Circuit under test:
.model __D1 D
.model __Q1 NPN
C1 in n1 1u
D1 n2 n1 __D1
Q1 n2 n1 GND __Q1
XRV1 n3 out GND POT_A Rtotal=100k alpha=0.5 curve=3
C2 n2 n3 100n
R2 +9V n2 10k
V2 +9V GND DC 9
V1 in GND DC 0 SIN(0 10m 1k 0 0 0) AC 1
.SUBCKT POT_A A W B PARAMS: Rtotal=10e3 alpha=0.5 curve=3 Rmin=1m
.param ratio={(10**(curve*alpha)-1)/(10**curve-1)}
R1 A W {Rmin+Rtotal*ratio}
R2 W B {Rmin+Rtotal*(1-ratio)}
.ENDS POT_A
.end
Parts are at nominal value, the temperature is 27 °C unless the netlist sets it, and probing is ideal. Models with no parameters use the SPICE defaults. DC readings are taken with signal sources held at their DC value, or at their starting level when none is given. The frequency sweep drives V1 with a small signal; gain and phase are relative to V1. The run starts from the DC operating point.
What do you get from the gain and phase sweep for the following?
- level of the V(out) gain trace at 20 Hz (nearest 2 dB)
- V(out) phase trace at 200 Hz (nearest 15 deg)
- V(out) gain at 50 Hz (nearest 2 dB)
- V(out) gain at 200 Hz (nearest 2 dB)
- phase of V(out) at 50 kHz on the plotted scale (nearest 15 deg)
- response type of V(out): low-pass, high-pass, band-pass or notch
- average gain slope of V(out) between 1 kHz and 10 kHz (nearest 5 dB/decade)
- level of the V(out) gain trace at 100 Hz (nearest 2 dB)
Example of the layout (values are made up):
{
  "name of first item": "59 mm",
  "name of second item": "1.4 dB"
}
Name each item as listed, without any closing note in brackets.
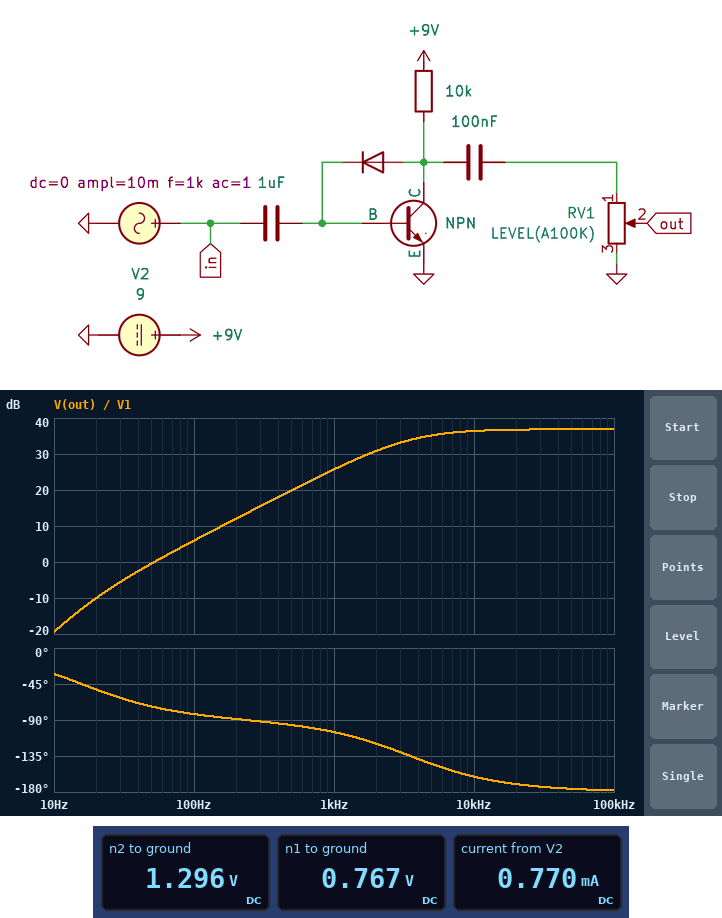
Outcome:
{
  "level of the V(out) gain trace at 20 Hz": "-10 dB",
  "V(out) phase trace at 200 Hz": "-90 deg",
  "V(out) gain at 50 Hz": "0 dB",
  "V(out) gain at 200 Hz": "12 dB",
  "phase of V(out) at 50 kHz on the plotted scale": "-180 deg",
  "response type of V(out): low-pass, high-pass, band-pass or notch": "high-pass",
  "average gain slope of V(out) between 1 kHz and 10 kHz": "10 dB/decade",
  "level of the V(out) gain trace at 100 Hz": "6 dB"
}
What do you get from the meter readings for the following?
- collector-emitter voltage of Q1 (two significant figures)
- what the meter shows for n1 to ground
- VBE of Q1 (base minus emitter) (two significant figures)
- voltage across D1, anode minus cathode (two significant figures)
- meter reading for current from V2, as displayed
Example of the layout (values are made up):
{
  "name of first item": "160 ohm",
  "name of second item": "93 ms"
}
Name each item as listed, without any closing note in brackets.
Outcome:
{
  "collector-emitter voltage of Q1": "1.3 V",
  "what the meter shows for n1 to ground": "0.767 V",
  "VBE of Q1 (base minus emitter)": "770 mV",
  "voltage across D1, anode minus cathode": "530 mV",
  "meter reading for current from V2, as displayed": "0.770 mA"
}
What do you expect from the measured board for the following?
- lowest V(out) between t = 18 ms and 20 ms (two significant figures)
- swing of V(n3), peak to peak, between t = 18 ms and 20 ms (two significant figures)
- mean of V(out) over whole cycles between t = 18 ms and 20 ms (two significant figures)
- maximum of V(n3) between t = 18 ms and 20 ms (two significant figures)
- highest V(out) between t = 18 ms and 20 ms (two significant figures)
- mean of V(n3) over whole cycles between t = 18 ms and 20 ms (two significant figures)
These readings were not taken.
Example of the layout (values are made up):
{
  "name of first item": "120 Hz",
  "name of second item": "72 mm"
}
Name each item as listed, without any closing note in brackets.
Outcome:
{
  "lowest V(out) between t = 18 ms and 20 ms": "-750 mV",
  "swing of V(n3), peak to peak, between t = 18 ms and 20 ms": "1.3 V",
  "mean of V(out) over whole cycles between t = 18 ms and 20 ms": "-77 mV",
  "maximum of V(n3) between t = 18 ms and 20 ms": "520 mV",
  "highest V(out) between t = 18 ms and 20 ms": "500 mV",
  "mean of V(n3) over whole cycles between t = 18 ms and 20 ms": "-79 mV"
}
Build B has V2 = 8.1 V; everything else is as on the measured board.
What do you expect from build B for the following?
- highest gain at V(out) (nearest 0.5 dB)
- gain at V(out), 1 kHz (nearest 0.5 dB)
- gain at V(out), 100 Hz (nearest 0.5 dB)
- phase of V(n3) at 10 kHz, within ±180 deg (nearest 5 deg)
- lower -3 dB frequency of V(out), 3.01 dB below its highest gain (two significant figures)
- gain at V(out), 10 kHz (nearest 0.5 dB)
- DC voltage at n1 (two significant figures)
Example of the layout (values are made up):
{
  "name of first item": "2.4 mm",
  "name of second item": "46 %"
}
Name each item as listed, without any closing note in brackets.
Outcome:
{
  "highest gain at V(out)": "36.5 dB",
  "gain at V(out), 1 kHz": "26.5 dB",
  "gain at V(out), 100 Hz": "7.0 dB",
  "phase of V(n3) at 10 kHz, within ±180 deg": "-165 deg",
  "lower -3 dB frequency of V(out), 3.01 dB below its highest gain": "3.0 kHz",
  "gain at V(out), 10 kHz": "36.0 dB",
  "DC voltage at n1": "760 mV"
}
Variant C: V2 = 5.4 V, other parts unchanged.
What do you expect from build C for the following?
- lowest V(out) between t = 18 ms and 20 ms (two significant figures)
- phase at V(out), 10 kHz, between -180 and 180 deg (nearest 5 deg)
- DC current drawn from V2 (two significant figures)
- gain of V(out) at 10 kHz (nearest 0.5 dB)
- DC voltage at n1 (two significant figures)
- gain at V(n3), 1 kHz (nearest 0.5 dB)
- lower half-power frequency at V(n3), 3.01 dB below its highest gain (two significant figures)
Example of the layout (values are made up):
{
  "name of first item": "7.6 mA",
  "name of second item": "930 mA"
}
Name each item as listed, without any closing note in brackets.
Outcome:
{
  "lowest V(out) between t = 18 ms and 20 ms": "-730 mV",
  "phase at V(out), 10 kHz, between -180 and 180 deg": "-170 deg",
  "DC current drawn from V2": "410 µA",
  "gain of V(out) at 10 kHz": "35.0 dB",
  "DC voltage at n1": "750 mV",
  "gain at V(n3), 1 kHz": "30.0 dB",
  "lower half-power frequency at V(n3), 3.01 dB below its highest gain": "1.5 kHz"
}
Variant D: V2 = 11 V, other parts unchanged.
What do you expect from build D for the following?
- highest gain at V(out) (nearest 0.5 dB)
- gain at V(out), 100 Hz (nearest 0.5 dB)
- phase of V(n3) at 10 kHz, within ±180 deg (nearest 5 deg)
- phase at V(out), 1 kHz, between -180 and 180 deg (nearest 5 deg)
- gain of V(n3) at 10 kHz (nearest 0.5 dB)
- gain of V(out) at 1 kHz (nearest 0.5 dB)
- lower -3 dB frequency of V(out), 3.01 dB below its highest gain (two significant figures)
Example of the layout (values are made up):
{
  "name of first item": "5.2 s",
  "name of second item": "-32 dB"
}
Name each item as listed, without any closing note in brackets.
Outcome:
{
  "highest gain at V(out)": "37.5 dB",
  "gain at V(out), 100 Hz": "4.0 dB",
  "phase of V(n3) at 10 kHz, within ±180 deg": "-155 deg",
  "phase at V(out), 1 kHz, between -180 and 180 deg": "-100 deg",
  "gain of V(n3) at 10 kHz": "37.0 dB",
  "gain of V(out) at 1 kHz": "24.0 dB",
  "lower -3 dB frequency of V(out), 3.01 dB below its highest gain": "4.6 kHz"
}
